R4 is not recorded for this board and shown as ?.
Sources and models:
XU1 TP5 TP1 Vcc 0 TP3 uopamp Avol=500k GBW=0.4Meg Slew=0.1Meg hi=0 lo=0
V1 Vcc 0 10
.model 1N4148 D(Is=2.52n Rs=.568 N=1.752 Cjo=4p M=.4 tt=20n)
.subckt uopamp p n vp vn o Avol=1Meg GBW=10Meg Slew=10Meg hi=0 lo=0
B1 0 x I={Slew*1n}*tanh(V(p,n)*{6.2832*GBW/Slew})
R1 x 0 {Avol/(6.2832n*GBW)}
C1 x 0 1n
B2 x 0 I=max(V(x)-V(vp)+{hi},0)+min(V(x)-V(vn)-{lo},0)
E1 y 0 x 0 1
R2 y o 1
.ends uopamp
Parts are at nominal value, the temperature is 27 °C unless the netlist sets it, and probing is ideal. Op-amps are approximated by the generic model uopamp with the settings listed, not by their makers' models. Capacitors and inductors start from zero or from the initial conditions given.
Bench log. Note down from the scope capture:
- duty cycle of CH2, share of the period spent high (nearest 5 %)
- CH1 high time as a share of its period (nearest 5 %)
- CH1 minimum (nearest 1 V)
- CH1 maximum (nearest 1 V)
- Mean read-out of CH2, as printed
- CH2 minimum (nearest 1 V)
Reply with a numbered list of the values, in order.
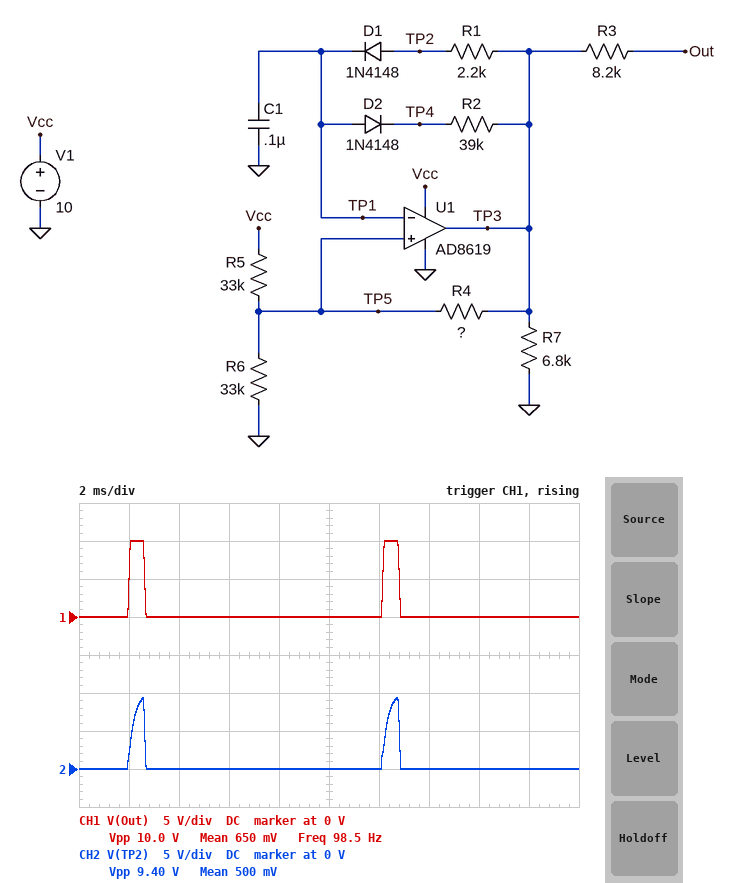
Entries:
1. 5 %
2. 5 %
3. 0 V
4. 10 V
5. 500 mV
6. 0 V
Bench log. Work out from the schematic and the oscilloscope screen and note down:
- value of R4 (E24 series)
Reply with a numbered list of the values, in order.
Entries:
1. 5.1 kΩ
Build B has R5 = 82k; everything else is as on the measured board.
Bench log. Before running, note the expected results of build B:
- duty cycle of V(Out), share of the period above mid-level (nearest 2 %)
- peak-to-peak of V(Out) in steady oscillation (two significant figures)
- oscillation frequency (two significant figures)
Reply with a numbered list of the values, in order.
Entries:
1. 4 %
2. 10 V
3. 60 Hz
